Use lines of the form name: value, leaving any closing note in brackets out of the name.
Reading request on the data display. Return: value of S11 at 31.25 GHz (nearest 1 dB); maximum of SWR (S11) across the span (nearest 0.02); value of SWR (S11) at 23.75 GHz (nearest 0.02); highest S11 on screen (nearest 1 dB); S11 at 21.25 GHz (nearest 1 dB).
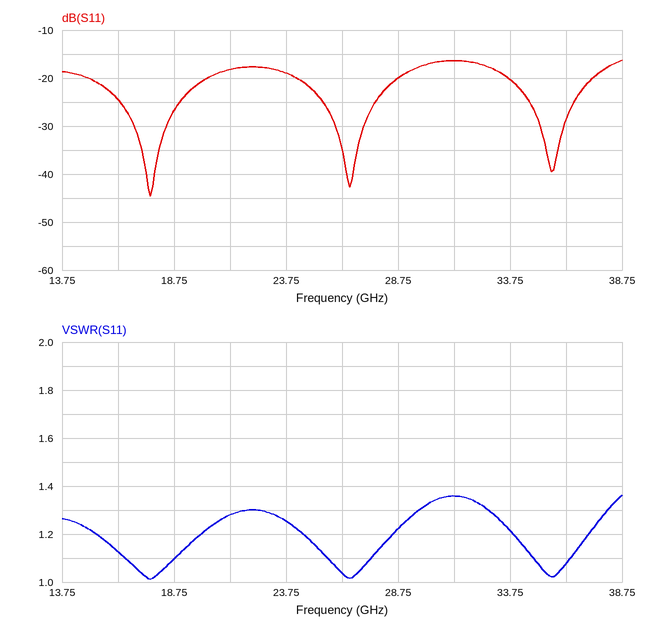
value of S11 at 31.25 GHz: -16 dB
maximum of SWR (S11) across the span: 1.36
value of SWR (S11) at 23.75 GHz: 1.26
highest S11 on screen: -16 dB
S11 at 21.25 GHz: -18 dB
